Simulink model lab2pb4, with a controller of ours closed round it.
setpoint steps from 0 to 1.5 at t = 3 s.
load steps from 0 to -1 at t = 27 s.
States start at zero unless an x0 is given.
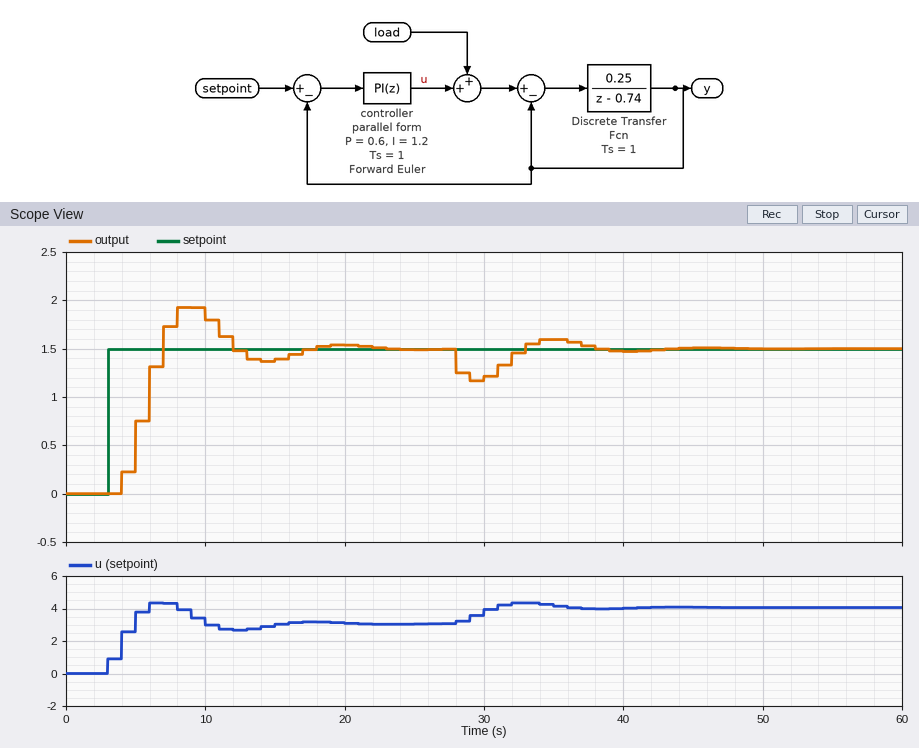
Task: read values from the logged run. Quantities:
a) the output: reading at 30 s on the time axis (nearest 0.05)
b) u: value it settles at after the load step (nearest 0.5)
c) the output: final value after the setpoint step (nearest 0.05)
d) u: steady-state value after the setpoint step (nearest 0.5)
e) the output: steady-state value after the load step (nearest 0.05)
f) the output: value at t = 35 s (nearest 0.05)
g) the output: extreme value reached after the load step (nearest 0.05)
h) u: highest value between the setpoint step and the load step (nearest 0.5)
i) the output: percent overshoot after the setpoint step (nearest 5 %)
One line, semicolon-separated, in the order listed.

1.20; 4.0; 1.50; 3.0; 1.50; 1.60; 1.15; 4.5; 30 %
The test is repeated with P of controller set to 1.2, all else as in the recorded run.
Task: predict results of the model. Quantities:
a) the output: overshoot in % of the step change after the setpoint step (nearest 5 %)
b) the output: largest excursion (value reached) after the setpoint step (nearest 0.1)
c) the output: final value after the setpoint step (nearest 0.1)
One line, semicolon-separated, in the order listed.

15 %; 1.7; 1.5
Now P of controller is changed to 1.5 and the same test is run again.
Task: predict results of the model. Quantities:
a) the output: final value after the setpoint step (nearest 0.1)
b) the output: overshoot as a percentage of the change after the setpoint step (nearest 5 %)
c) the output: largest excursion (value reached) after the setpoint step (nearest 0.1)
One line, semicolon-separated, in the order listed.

1.5; 10 %; 1.6
